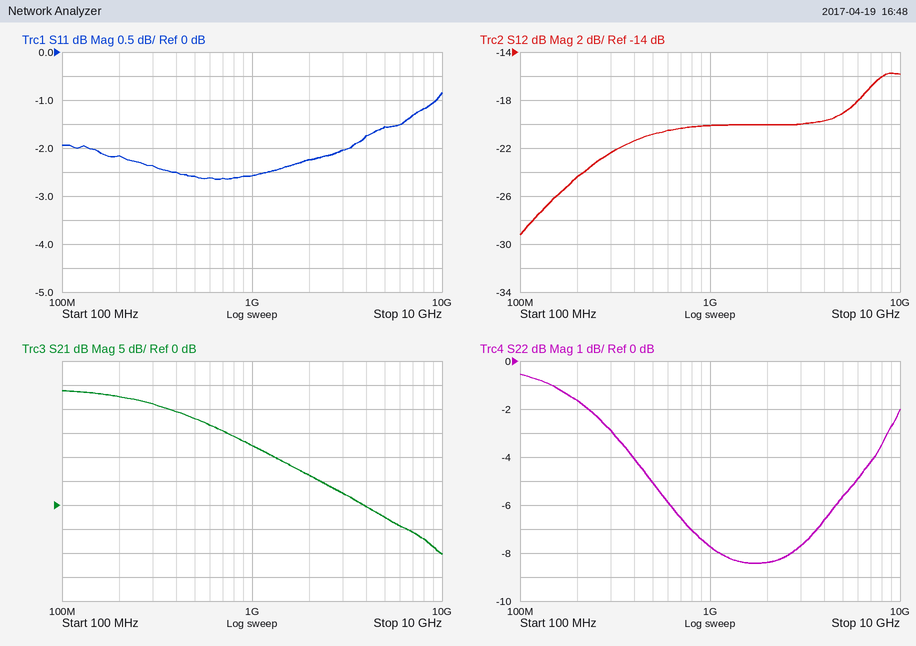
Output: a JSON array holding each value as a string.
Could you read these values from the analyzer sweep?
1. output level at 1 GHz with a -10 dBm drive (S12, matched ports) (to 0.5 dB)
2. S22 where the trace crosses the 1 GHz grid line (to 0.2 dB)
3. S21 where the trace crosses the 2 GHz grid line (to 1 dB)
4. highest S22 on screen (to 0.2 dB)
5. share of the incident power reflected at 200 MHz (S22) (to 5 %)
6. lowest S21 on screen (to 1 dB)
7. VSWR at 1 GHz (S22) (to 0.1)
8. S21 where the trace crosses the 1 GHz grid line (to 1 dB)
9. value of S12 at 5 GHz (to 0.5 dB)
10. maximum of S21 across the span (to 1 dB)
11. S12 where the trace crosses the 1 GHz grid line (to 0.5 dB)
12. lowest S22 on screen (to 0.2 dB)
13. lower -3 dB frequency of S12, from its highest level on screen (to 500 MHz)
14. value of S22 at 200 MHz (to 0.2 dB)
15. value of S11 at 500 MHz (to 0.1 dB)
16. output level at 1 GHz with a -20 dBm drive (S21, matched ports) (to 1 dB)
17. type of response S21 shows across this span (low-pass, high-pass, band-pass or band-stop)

["-30.0 dBm", "-7.8 dB", "6 dB", "-0.6 dB", "70 %", "-10 dB", "2.4", "12 dB", "-19.0 dB", "24 dB", "-20.0 dB", "-8.4 dB", "5.5 GHz", "-1.6 dB", "-2.6 dB", "-8 dBm", "low-pass"]
